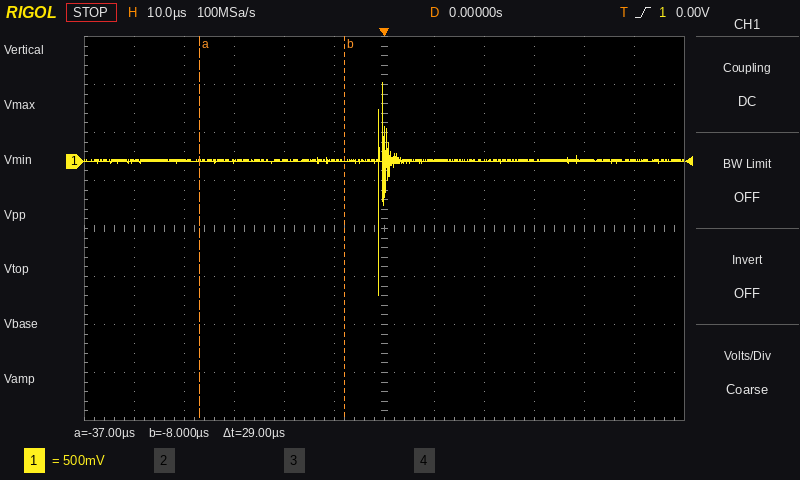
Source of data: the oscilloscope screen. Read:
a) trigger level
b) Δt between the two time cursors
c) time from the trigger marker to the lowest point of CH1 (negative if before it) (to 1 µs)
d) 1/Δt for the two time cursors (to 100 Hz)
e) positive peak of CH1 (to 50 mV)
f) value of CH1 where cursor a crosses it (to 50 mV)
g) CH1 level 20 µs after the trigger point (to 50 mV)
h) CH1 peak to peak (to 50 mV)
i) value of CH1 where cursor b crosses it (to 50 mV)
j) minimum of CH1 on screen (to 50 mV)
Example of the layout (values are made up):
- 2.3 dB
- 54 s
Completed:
- 0.00 V
- 29 µs
- -1 µs
- 34.5 kHz
- 800 mV
- 0 mV
- 0 mV
- 2.20 V
- 0 mV
- -1.40 V
